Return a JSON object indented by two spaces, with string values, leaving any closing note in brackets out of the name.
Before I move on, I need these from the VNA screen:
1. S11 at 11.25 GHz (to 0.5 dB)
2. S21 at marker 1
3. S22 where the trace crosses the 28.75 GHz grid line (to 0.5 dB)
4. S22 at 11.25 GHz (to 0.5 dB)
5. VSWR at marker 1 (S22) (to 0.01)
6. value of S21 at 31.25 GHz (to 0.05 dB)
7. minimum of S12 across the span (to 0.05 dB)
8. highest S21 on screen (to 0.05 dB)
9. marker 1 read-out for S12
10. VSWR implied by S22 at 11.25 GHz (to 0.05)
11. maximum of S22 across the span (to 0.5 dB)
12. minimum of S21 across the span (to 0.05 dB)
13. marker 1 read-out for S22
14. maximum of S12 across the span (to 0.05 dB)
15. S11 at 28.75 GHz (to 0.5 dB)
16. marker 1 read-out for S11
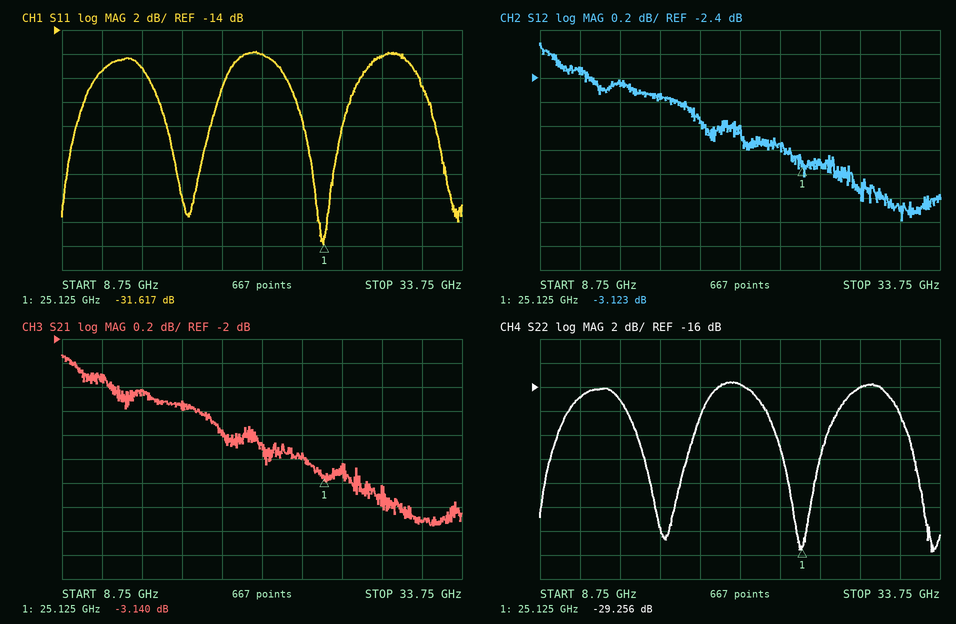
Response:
{
  "S11 at 11.25 GHz": "-17.5 dB",
  "S21 at marker 1": "-3.140 dB",
  "S22 where the trace crosses the 28.75 GHz grid line": "-16.0 dB",
  "S22 at 11.25 GHz": "-17.0 dB",
  "VSWR at marker 1 (S22)": "1.07",
  "value of S21 at 31.25 GHz": "-3.50 dB",
  "minimum of S12 across the span": "-3.60 dB",
  "highest S21 on screen": "-2.15 dB",
  "marker 1 read-out for S12": "-3.123 dB",
  "VSWR implied by S22 at 11.25 GHz": "1.35",
  "maximum of S22 across the span": "-15.5 dB",
  "minimum of S21 across the span": "-3.55 dB",
  "marker 1 read-out for S22": "-29.256 dB",
  "maximum of S12 across the span": "-2.10 dB",
  "S11 at 28.75 GHz": "-16.0 dB",
  "marker 1 read-out for S11": "-31.617 dB"
}
